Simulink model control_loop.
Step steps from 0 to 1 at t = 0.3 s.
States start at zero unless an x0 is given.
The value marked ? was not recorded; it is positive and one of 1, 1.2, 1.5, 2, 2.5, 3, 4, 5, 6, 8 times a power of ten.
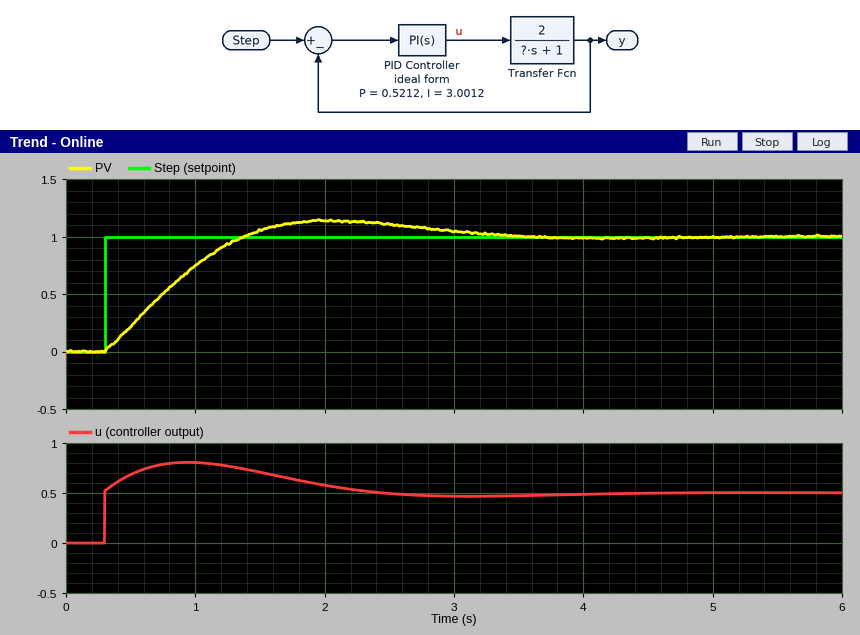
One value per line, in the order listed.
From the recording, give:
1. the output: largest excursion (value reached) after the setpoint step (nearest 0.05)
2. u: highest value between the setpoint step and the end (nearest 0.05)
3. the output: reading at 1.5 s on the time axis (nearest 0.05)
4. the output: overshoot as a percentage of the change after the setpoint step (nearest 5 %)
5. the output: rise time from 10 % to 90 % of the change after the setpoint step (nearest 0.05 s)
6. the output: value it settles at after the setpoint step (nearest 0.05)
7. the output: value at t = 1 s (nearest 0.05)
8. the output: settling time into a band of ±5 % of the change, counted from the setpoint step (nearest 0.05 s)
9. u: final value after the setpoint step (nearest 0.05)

1.15
0.80
1.05
15 %
0.80 s
1.00
0.75
2.65 s
0.50
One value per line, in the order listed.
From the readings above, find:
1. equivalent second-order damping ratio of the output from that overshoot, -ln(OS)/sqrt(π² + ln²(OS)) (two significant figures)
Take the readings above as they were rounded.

0.52
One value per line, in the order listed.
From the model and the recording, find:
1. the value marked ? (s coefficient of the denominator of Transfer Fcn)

1
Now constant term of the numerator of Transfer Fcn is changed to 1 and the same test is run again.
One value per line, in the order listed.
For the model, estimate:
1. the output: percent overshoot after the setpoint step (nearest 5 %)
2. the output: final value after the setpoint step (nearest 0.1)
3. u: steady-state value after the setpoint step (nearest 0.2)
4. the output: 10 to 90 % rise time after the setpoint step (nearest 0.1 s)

10 %
1.0
1.0
1.3 s
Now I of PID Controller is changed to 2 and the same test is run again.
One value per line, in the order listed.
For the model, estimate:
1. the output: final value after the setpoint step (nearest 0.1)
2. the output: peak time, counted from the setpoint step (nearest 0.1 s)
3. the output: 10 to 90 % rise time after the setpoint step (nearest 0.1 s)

1.0
2.3 s
1.1 s
